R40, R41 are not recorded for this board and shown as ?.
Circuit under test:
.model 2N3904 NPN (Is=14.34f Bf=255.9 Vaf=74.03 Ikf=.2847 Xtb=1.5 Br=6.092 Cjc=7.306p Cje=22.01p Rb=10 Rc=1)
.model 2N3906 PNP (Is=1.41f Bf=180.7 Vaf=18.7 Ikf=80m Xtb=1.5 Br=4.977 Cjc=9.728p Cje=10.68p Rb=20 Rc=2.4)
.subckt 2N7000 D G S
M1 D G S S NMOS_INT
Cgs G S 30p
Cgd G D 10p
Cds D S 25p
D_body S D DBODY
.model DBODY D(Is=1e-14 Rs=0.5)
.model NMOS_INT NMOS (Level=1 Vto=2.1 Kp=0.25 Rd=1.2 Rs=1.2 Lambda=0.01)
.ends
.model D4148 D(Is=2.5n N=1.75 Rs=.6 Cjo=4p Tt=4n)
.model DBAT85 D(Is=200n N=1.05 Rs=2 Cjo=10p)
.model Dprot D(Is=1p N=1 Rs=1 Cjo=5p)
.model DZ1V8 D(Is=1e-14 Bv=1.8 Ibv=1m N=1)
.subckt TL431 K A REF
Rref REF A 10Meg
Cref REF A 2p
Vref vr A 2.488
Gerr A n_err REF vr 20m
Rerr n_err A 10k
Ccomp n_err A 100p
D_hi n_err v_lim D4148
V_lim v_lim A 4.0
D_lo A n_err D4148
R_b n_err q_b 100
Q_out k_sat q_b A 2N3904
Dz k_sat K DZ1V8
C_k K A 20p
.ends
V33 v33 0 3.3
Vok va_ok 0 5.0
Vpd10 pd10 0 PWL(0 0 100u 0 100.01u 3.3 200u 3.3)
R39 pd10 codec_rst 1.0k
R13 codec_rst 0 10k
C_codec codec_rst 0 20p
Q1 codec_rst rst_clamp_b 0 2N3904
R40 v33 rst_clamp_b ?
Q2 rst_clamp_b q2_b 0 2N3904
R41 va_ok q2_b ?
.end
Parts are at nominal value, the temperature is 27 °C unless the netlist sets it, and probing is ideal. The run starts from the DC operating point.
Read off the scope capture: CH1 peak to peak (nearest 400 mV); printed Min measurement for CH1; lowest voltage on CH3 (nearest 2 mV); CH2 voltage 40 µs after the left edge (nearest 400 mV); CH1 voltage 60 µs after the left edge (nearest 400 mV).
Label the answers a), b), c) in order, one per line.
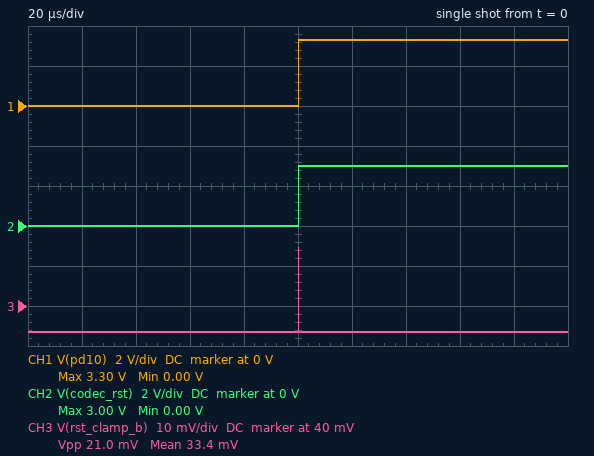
a) 3.2 V
b) 0.00 V
c) 34 mV
d) 0 V
e) 0 V
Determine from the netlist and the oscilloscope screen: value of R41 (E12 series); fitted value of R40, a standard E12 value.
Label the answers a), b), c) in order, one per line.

a) 68 kΩ
b) 3.9 kΩ
